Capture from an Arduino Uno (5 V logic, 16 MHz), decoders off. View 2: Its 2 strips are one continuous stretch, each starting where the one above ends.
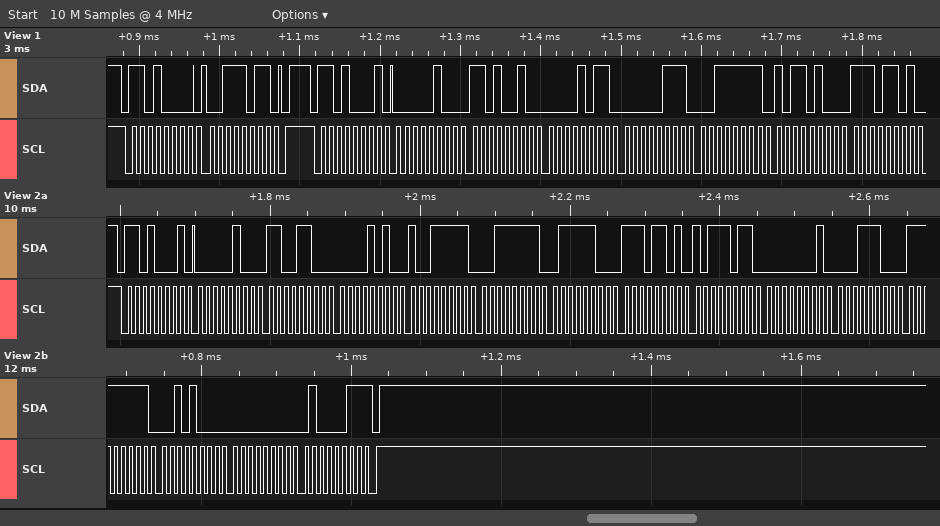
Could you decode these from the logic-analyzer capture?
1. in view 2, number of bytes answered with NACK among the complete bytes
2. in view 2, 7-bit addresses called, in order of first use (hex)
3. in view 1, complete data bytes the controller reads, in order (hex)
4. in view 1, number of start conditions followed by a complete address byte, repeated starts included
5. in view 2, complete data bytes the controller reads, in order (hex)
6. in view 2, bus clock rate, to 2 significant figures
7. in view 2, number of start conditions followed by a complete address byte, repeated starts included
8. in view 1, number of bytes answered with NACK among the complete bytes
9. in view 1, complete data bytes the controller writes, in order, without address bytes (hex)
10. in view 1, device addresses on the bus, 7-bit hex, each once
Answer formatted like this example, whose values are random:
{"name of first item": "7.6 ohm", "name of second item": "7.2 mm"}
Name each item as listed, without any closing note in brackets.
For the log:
{"in view 2, number of bytes answered with NACK among the complete bytes": "1", "in view 2, 7-bit addresses called, in order of first use": "0x68", "in view 1, complete data bytes the controller reads, in order": "04 D2 0B 07 3F B4 ED", "in view 1, number of start conditions followed by a complete address byte, repeated starts included": "2", "in view 2, complete data bytes the controller reads, in order": "04 CC 0A 9F 3F 7C ED BB 01 1C FF 28 00 43", "in view 2, bus clock rate, to 2 significant figures": "100 kHz", "in view 2, number of start conditions followed by a complete address byte, repeated starts included": "1", "in view 1, number of bytes answered with NACK among the complete bytes": "0", "in view 1, complete data bytes the controller writes, in order, without address bytes": "3B", "in view 1, device addresses on the bus, 7-bit hex, each once": "0x68"}
